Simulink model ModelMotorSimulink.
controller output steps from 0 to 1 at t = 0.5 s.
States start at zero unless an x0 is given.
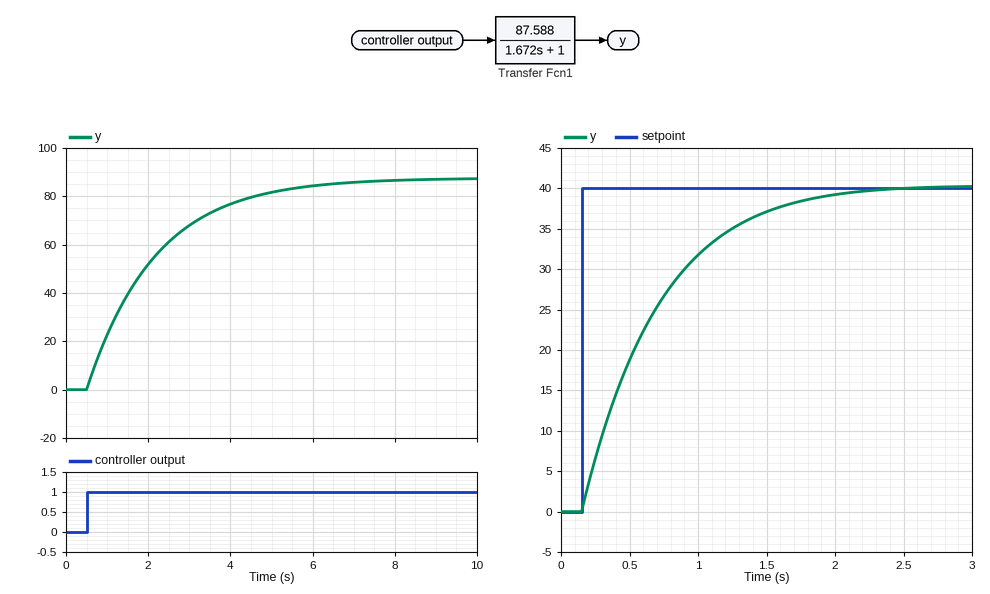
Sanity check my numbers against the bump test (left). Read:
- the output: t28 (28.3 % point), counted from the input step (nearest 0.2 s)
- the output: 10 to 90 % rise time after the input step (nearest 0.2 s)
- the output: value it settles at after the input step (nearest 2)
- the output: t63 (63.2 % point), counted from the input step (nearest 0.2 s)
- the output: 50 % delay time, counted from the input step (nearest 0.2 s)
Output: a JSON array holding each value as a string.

["0.6 s", "3.6 s", "88", "1.6 s", "1.2 s"]
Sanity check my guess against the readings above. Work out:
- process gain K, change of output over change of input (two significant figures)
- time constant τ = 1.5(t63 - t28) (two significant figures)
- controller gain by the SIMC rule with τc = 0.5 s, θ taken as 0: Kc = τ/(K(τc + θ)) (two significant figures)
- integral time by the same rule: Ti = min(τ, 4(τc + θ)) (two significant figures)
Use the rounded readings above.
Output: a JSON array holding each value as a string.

["88", "1.5 s", "0.034", "1.5 s"]
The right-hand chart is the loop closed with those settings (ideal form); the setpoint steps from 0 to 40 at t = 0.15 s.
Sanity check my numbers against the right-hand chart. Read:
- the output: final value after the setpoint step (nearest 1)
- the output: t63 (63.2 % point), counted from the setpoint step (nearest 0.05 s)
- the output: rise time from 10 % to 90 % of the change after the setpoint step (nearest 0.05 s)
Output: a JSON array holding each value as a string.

["40", "0.55 s", "1.15 s"]
